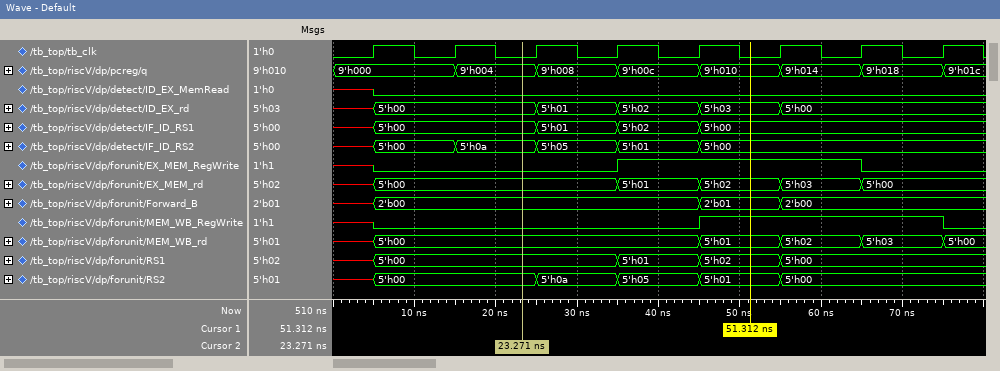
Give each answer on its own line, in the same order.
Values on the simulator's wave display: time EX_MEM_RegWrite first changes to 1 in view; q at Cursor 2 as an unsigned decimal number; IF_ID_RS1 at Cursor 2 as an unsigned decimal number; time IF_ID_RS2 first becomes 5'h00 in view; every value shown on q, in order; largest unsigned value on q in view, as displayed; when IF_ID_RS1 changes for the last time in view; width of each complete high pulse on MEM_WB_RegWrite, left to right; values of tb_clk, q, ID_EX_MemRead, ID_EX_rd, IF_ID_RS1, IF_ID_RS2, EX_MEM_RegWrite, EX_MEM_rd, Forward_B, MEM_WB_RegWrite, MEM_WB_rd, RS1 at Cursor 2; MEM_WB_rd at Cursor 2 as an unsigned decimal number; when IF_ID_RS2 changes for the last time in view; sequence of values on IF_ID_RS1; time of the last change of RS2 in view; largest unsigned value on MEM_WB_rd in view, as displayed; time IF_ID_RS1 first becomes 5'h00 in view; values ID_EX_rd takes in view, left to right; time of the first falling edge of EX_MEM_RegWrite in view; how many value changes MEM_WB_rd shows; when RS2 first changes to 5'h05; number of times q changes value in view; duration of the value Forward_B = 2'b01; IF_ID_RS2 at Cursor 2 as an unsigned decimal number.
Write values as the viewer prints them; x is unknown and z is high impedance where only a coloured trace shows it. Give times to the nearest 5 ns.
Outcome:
35 ns
4
0
5 ns
9'h000, 9'h004, 9'h008, 9'h00c, 9'h010, 9'h014, 9'h018, 9'h01c
9'h01c
45 ns
30 ns
tb_clk=0, q=9'h004, ID_EX_MemRead=0, ID_EX_rd=5'h00, IF_ID_RS1=5'h00, IF_ID_RS2=5'h0a, EX_MEM_RegWrite=0, EX_MEM_rd=5'h00, Forward_B=2'b00, MEM_WB_RegWrite=0, MEM_WB_rd=5'h00, RS1=5'h00
0
45 ns
x, 5'h00, 5'h01, 5'h02, 5'h00
55 ns
5'h03
5 ns
x, 5'h00, 5'h01, 5'h02, 5'h03, 5'h00
65 ns
5
35 ns
7
10 ns
10
